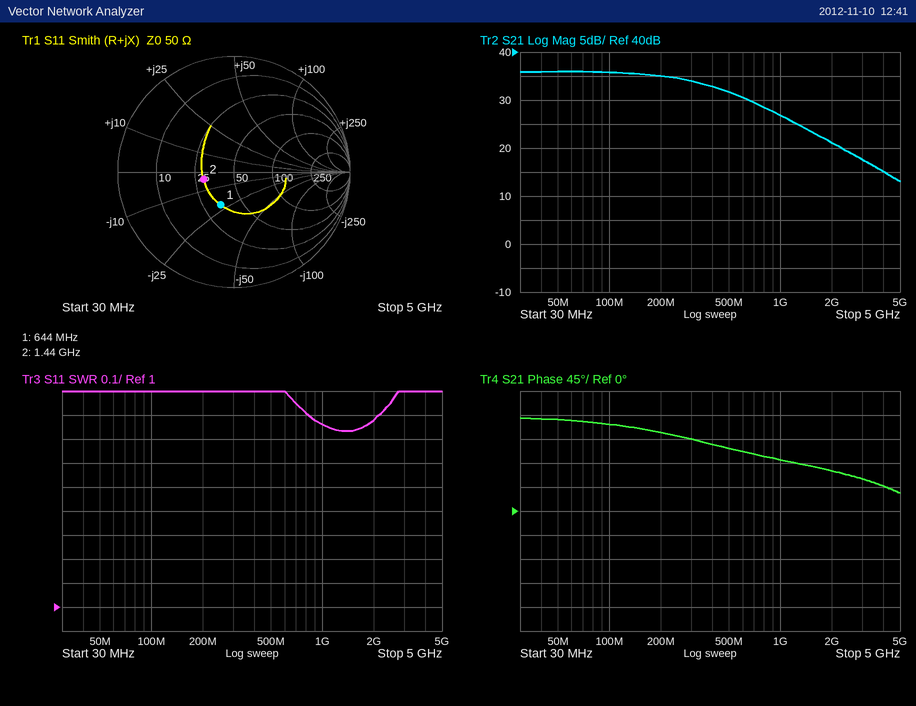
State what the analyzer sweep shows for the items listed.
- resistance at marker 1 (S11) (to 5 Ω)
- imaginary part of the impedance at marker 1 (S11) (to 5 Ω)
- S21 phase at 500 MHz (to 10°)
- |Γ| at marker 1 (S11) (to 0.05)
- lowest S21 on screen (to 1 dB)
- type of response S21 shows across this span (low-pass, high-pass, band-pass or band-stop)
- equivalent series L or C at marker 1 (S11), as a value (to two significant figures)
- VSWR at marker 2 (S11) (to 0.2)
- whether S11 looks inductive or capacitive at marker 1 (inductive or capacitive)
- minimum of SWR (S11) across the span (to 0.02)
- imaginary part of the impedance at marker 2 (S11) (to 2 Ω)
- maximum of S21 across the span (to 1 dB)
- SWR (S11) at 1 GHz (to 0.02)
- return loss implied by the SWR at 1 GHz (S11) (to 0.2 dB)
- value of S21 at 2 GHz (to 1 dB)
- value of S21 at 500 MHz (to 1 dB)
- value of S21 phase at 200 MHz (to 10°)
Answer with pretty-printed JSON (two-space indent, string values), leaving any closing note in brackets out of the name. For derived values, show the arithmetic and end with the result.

{
  "resistance at marker 1 (S11)": "35 Ω",
  "imaginary part of the impedance at marker 1 (S11)": "-20 Ω",
  "S21 phase at 500 MHz": "120°",
  "|Γ| at marker 1 (S11)": "0.30",
  "lowest S21 on screen": "13 dB",
  "type of response S21 shows across this span": "low-pass",
  "equivalent series L or C at marker 1 (S11), as a value": "C = 1/(2π × 644 MHz × 20 Ω) ≈ 12 pF",
  "VSWR at marker 2 (S11)": "1.8",
  "whether S11 looks inductive or capacitive at marker 1": "capacitive",
  "minimum of SWR (S11) across the span": "1.74",
  "imaginary part of the impedance at marker 2 (S11)": "-4 Ω",
  "maximum of S21 across the span": "36 dB",
  "SWR (S11) at 1 GHz": "1.76",
  "return loss implied by the SWR at 1 GHz (S11)": "−20 log10((1.76 − 1)/(1.76 + 1)) ≈ 11.2 dB",
  "value of S21 at 2 GHz": "21 dB",
  "value of S21 at 500 MHz": "32 dB",
  "value of S21 phase at 200 MHz": "150°"
}
